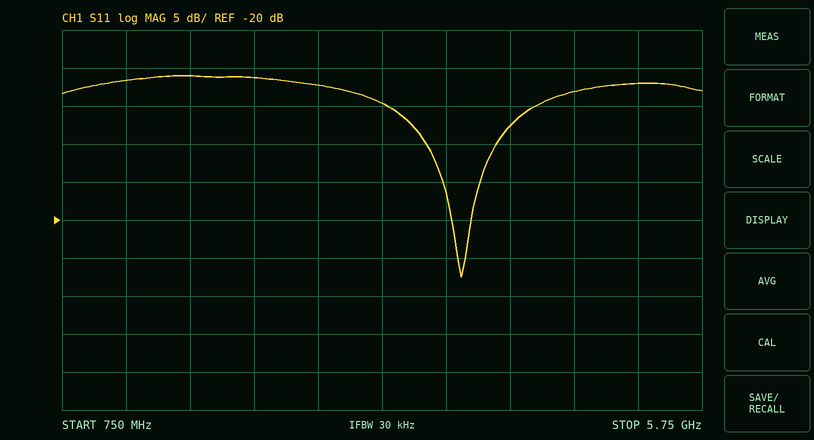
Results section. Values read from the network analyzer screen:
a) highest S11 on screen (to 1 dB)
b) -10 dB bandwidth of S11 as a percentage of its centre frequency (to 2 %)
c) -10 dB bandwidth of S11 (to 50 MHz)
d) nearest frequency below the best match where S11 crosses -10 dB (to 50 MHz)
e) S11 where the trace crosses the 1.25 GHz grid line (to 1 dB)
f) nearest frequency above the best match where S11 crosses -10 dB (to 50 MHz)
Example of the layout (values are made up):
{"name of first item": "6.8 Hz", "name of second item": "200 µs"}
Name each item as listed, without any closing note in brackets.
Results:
{"highest S11 on screen": "-1 dB", "-10 dB bandwidth of S11 as a percentage of its centre frequency": "14 %", "-10 dB bandwidth of S11": "550 MHz", "nearest frequency below the best match where S11 crosses -10 dB": "3.60 GHz", "S11 where the trace crosses the 1.25 GHz grid line": "-2 dB", "nearest frequency above the best match where S11 crosses -10 dB": "4.15 GHz"}
